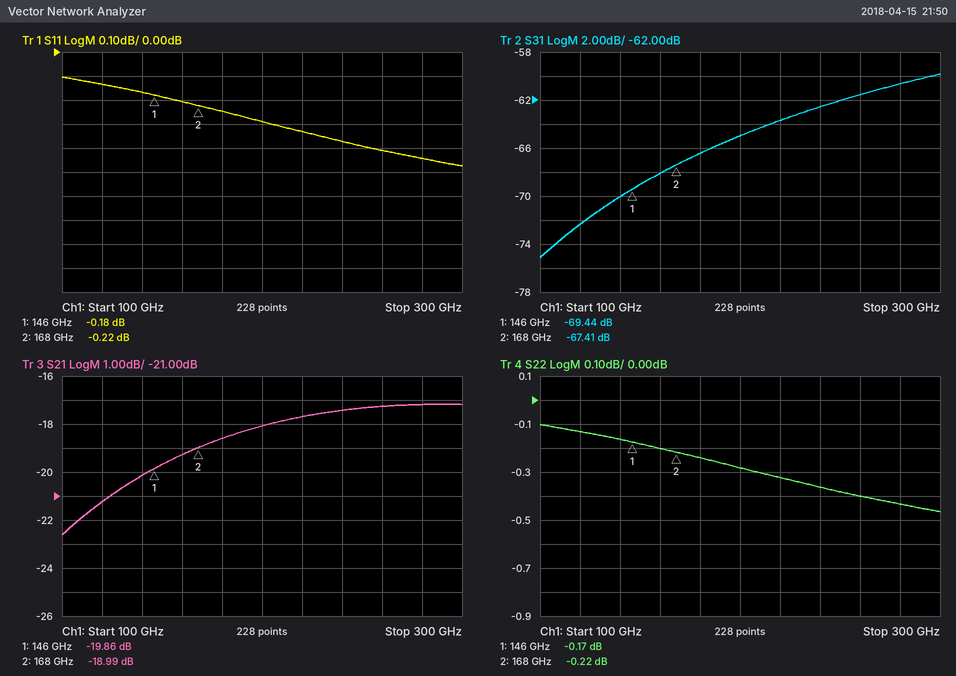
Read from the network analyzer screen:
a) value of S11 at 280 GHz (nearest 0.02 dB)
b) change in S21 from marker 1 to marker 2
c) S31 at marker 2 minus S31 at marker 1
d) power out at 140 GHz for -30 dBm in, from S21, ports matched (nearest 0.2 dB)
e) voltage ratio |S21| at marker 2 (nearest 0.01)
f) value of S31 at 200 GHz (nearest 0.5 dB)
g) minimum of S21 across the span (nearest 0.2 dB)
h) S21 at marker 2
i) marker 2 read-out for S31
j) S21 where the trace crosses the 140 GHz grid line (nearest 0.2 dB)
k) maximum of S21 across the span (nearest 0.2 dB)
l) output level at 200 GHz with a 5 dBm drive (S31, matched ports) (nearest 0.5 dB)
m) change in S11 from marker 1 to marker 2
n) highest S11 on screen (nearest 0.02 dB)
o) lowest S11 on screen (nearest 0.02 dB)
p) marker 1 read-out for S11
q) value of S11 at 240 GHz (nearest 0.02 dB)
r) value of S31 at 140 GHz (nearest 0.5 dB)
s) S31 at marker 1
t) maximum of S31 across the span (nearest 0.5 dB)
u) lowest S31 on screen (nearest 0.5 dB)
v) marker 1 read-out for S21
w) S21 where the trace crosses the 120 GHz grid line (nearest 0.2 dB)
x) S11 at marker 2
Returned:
-0.44 dB
0.87 dB
2.03 dB
-50.2 dBm
0.11
-65.0 dB
-22.6 dB
-18.99 dB
-67.41 dB
-20.2 dB
-17.2 dB
-60.0 dBm
-0.04 dB
-0.10 dB
-0.48 dB
-0.18 dB
-0.38 dB
-70.0 dB
-69.44 dB
-60.0 dB
-75.0 dB
-19.86 dB
-21.2 dB
-0.22 dB
